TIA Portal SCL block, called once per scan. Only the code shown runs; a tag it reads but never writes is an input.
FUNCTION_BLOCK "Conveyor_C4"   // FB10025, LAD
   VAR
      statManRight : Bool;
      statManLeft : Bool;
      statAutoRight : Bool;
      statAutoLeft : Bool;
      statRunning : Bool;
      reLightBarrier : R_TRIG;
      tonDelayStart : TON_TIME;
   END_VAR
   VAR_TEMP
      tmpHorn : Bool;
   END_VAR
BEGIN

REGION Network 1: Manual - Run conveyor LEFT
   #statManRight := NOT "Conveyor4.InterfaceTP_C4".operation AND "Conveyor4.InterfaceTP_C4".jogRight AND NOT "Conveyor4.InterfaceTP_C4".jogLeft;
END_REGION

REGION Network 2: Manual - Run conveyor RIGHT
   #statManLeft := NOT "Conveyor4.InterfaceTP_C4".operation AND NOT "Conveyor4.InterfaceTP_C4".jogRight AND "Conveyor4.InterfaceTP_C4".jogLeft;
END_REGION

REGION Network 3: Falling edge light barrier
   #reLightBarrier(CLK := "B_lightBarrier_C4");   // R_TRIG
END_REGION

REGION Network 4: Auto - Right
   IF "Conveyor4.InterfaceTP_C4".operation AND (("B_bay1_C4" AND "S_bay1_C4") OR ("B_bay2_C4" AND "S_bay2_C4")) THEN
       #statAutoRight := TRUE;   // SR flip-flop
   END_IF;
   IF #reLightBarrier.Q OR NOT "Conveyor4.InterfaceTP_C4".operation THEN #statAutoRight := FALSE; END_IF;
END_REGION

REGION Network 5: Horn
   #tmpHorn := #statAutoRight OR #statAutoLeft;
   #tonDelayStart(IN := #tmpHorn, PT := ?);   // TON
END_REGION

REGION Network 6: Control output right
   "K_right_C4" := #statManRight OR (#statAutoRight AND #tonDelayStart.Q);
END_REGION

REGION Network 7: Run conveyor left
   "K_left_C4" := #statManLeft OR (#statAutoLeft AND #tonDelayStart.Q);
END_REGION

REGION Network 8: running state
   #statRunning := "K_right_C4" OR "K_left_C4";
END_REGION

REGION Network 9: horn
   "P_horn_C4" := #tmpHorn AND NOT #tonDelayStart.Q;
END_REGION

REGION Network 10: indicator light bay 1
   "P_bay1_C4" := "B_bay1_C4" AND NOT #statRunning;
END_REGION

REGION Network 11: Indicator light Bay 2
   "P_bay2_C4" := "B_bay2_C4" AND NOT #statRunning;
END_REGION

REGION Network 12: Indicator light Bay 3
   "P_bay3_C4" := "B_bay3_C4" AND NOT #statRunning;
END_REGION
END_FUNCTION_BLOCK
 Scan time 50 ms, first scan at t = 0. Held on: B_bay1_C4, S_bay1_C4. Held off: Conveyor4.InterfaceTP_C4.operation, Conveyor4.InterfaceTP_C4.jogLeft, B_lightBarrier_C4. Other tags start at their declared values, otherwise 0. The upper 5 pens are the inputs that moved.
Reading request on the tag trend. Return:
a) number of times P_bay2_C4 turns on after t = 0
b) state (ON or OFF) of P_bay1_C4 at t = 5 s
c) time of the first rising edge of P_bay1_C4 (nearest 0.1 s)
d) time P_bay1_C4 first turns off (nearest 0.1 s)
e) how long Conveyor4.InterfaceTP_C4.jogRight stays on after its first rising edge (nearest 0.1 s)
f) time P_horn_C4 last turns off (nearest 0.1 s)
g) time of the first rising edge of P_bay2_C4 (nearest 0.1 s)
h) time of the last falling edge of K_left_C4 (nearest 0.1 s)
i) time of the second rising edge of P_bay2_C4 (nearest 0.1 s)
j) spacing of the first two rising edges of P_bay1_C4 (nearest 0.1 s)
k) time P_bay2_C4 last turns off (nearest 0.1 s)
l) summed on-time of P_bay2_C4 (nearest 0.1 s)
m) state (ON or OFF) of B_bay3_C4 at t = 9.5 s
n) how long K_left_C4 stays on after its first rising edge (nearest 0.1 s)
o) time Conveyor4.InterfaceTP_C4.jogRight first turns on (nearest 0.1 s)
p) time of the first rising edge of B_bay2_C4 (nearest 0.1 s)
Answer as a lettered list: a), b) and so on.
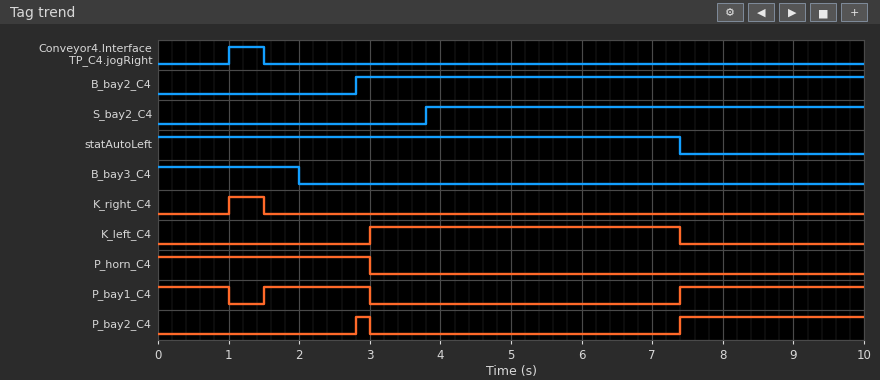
a) 2
b) OFF
c) 1.5 s
d) 1.0 s
e) 0.5 s
f) 3.0 s
g) 2.8 s
h) 7.4 s
i) 7.4 s
j) 5.9 s
k) 3.0 s
l) 2.8 s
m) OFF
n) 4.4 s
o) 1.0 s
p) 2.8 s
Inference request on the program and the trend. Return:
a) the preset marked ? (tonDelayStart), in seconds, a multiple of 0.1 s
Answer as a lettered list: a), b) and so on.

a) 3.0 s
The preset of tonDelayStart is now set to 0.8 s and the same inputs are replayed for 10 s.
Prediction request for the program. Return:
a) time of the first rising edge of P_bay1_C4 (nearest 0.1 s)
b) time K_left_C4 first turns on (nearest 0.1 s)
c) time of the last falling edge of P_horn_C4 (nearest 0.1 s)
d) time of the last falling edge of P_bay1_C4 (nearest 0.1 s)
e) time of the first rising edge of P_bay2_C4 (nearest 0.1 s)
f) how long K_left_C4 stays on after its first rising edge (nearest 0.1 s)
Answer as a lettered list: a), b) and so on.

a) 7.4 s
b) 0.8 s
c) 0.8 s
d) 0.8 s
e) 7.4 s
f) 6.6 s
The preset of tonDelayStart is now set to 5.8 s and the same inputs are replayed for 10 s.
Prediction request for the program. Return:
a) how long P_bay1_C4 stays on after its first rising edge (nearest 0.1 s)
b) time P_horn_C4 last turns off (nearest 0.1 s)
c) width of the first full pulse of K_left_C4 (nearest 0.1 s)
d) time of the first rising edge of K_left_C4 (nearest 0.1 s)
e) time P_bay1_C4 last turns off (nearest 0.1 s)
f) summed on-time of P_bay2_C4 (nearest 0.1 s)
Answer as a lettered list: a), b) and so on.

a) 4.3 s
b) 5.8 s
c) 1.6 s
d) 5.8 s
e) 5.8 s
f) 5.6 s
